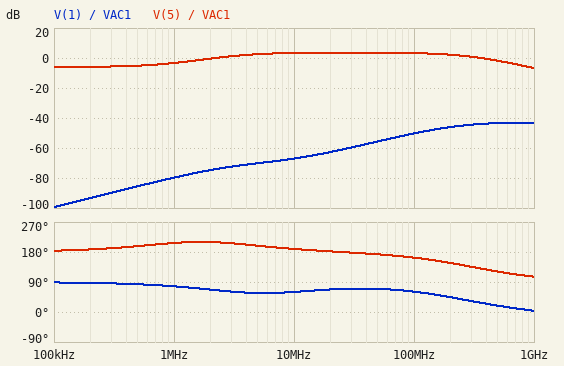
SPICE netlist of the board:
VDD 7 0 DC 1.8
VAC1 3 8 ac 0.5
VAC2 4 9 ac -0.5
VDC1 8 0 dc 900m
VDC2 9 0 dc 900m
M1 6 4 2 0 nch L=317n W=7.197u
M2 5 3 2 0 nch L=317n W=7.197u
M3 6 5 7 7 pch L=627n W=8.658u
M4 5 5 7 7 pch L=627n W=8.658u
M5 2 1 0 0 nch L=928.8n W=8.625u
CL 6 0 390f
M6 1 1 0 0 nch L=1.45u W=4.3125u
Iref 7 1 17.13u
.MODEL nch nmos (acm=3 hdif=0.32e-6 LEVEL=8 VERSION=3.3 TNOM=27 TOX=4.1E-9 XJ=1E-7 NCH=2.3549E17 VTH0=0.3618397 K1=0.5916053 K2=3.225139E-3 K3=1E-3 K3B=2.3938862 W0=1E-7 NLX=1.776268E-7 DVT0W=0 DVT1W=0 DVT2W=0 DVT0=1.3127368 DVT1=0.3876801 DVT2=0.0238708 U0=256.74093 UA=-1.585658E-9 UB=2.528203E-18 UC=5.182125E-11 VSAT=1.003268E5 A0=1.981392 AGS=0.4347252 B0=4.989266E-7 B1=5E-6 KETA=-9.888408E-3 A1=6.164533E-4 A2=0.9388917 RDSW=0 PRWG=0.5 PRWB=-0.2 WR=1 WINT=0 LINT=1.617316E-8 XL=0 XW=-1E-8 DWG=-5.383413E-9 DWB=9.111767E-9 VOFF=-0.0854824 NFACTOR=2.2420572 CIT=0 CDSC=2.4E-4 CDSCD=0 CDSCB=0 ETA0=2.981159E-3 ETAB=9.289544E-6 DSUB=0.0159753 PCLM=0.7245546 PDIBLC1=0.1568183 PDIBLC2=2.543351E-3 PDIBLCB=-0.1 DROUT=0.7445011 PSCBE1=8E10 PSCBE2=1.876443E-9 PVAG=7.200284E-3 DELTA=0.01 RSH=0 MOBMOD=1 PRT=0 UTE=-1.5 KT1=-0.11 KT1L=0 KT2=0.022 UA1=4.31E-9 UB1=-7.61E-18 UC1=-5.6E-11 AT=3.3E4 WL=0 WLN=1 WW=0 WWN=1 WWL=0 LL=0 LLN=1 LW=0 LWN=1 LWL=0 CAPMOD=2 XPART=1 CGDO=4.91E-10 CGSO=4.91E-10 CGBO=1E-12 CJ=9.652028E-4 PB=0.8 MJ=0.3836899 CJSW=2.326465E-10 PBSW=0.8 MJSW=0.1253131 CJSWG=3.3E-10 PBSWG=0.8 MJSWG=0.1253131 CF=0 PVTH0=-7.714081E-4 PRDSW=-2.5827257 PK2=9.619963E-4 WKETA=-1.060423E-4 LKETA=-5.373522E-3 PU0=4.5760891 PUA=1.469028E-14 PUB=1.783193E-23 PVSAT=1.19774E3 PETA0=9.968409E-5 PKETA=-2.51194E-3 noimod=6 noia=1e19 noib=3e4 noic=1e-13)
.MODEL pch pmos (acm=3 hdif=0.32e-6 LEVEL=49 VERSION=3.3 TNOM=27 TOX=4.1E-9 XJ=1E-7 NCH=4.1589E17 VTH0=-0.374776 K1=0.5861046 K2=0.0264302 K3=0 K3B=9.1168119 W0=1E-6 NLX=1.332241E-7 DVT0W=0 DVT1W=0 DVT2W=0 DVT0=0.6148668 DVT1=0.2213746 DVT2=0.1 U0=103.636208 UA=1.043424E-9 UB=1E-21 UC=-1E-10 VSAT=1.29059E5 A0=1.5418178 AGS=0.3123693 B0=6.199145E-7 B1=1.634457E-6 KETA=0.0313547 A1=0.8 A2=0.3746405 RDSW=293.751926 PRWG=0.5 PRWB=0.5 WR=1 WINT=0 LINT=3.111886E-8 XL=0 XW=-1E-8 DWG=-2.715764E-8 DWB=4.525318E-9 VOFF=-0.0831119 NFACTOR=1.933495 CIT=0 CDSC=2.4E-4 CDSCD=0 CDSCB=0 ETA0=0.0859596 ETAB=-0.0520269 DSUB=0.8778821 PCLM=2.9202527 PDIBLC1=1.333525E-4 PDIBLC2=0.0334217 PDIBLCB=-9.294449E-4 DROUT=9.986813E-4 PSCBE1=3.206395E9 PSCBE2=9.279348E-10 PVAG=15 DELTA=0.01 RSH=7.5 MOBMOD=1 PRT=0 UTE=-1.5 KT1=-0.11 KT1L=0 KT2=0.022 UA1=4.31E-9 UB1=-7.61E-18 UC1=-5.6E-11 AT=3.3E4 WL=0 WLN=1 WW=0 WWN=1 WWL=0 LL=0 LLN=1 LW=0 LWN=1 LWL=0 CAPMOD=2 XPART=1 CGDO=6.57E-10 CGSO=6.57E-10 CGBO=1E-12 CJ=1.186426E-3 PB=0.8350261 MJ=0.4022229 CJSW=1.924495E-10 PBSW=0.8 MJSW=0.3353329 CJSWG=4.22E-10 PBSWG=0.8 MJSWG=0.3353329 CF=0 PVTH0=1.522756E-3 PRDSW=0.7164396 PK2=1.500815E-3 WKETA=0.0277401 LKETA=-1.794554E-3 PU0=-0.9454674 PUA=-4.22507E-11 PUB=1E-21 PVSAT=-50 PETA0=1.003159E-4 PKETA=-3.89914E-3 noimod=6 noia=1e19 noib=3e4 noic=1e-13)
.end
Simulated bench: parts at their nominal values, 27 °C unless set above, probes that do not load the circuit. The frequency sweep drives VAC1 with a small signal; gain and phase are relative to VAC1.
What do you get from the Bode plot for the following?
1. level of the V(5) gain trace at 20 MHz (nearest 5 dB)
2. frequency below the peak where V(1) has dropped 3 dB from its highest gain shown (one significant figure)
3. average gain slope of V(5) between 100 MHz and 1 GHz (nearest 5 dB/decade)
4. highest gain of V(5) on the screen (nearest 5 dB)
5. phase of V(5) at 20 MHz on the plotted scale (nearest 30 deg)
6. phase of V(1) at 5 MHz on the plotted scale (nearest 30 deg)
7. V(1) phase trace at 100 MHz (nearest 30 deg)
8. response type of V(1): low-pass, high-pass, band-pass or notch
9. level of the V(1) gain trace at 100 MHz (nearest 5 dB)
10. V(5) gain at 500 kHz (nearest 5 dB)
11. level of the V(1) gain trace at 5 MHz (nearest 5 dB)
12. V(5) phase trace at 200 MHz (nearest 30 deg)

5 dB
200 MHz
-10 dB/decade
5 dB
180 deg
60 deg
60 deg
high-pass
-50 dB
-5 dB
-70 dB
150 deg
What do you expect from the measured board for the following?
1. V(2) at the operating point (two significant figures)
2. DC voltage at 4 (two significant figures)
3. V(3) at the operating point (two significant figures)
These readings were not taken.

280 mV
900 mV
900 mV
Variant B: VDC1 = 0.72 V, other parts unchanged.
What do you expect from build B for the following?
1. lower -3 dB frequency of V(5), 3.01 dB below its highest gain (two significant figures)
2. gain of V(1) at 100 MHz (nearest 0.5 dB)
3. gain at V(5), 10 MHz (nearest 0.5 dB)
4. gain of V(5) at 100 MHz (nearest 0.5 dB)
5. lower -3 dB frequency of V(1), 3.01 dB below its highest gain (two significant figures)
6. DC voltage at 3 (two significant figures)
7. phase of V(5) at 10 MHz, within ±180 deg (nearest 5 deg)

120 MHz
-34.0 dB
-15.0 dB
-3.5 dB
92 MHz
720 mV
-160 deg
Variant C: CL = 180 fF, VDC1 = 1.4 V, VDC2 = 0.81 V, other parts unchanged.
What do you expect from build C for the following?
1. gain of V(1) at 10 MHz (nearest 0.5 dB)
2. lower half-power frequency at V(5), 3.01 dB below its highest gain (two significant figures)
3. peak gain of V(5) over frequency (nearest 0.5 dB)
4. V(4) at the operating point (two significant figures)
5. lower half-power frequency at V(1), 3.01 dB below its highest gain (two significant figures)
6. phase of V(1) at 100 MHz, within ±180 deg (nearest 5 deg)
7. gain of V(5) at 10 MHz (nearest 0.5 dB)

-57.5 dB
240 MHz
-14.5 dB
810 mV
190 MHz
65 deg
-37.0 dB
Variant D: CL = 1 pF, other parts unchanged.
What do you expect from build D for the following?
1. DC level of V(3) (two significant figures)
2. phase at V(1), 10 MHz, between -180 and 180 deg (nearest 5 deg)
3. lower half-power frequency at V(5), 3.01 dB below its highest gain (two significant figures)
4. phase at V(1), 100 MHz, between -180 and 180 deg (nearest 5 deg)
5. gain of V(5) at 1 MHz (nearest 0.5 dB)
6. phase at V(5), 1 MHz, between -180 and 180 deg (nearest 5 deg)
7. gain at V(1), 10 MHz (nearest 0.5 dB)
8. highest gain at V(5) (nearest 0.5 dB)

900 mV
75 deg
1.1 MHz
65 deg
0.5 dB
-150 deg
-69.0 dB
4.0 dB
